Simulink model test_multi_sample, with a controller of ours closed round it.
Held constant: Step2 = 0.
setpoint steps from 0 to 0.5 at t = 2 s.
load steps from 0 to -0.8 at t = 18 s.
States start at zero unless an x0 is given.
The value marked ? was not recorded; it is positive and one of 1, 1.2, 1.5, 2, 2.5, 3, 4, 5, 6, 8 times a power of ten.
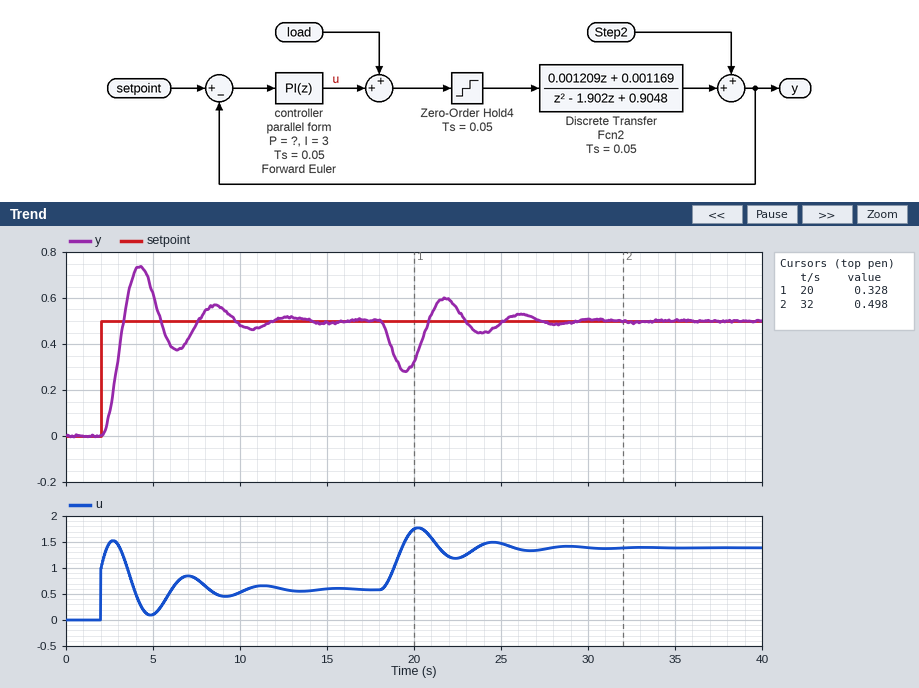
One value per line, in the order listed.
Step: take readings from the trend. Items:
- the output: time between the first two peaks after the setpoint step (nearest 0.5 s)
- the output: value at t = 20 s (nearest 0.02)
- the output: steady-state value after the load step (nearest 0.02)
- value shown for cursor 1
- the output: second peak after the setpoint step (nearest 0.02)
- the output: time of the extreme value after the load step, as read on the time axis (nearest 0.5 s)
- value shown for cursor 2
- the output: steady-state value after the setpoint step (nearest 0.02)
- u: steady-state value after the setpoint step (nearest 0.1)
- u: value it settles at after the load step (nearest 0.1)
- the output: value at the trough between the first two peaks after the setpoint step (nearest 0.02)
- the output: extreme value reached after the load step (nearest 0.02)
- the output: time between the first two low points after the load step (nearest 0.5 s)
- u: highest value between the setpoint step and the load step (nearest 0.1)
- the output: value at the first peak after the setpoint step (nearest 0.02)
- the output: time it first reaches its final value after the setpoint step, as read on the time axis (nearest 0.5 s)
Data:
4.5 s
0.32
0.50
0.328
0.56
19.5 s
0.498
0.50
0.6
1.4
0.38
0.28
4.5 s
1.5
0.74
3.5 s
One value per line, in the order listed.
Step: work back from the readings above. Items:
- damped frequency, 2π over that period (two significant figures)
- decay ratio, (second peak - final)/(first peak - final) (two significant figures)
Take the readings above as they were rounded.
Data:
1.4 rad/s
0.25
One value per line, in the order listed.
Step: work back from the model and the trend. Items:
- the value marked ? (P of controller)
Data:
2
